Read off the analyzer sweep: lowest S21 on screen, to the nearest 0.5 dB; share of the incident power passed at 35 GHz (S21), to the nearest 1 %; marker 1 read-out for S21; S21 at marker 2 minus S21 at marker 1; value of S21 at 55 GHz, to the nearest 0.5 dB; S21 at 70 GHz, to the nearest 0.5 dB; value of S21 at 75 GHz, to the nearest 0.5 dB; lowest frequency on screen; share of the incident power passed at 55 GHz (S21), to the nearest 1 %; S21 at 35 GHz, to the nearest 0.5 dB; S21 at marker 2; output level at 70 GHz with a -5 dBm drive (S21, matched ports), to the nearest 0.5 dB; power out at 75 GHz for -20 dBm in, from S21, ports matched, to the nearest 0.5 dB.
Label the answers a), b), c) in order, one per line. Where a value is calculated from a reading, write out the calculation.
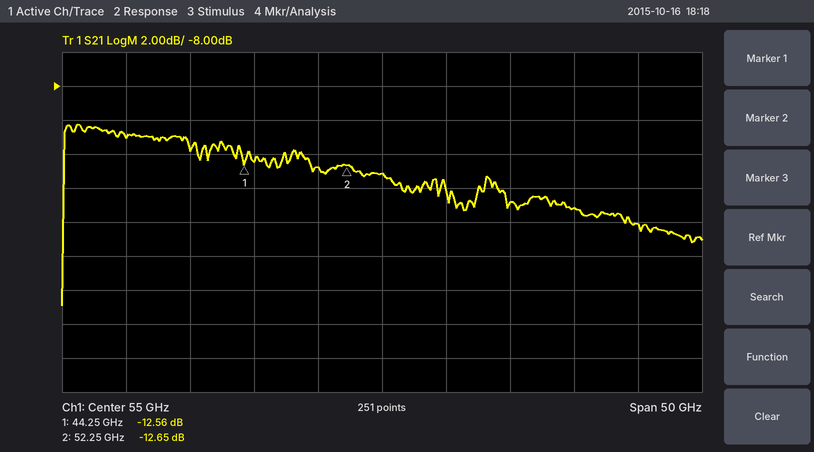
a) -21.0 dB
b) 10^(-11/10) ≈ 8 %
c) -12.56 dB
d) -12.65 − (-12.56) = -0.09 dB
e) -13.0 dB
f) -15.0 dB
g) -16.0 dB
h) 30 GHz
i) 10^(-13/10) ≈ 5 %
j) -11.0 dB
k) -12.65 dB
l) -5 dBm + (-15.0 dB) = -20.0 dBm
m) -20 dBm + (-16.0 dB) = -36.0 dBm
